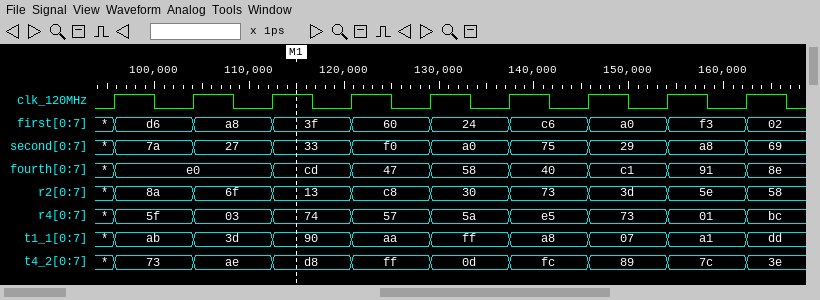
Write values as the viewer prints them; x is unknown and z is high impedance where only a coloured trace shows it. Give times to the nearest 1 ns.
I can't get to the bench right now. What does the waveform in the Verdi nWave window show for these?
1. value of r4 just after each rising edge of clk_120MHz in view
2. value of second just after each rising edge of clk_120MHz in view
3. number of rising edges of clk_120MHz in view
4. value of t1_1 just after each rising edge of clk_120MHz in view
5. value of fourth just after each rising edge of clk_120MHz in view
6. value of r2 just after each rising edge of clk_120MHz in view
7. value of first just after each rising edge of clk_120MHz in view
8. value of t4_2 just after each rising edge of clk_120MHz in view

5f, 03, 74, 57, 5a, e5, 73, 01, bc
7a, 27, 33, f0, a0, 75, 29, a8, 69
9
ab, 3d, 90, aa, ff, a8, 07, a1, dd
e0, e0, cd, 47, 58, 40, c1, 91, 8e
8a, 6f, 13, c8, 30, 73, 3d, 5e, 58
d6, a8, 3f, 60, 24, c6, a0, f3, 02
73, ae, d8, ff, 0d, fc, 89, 7c, 3e
